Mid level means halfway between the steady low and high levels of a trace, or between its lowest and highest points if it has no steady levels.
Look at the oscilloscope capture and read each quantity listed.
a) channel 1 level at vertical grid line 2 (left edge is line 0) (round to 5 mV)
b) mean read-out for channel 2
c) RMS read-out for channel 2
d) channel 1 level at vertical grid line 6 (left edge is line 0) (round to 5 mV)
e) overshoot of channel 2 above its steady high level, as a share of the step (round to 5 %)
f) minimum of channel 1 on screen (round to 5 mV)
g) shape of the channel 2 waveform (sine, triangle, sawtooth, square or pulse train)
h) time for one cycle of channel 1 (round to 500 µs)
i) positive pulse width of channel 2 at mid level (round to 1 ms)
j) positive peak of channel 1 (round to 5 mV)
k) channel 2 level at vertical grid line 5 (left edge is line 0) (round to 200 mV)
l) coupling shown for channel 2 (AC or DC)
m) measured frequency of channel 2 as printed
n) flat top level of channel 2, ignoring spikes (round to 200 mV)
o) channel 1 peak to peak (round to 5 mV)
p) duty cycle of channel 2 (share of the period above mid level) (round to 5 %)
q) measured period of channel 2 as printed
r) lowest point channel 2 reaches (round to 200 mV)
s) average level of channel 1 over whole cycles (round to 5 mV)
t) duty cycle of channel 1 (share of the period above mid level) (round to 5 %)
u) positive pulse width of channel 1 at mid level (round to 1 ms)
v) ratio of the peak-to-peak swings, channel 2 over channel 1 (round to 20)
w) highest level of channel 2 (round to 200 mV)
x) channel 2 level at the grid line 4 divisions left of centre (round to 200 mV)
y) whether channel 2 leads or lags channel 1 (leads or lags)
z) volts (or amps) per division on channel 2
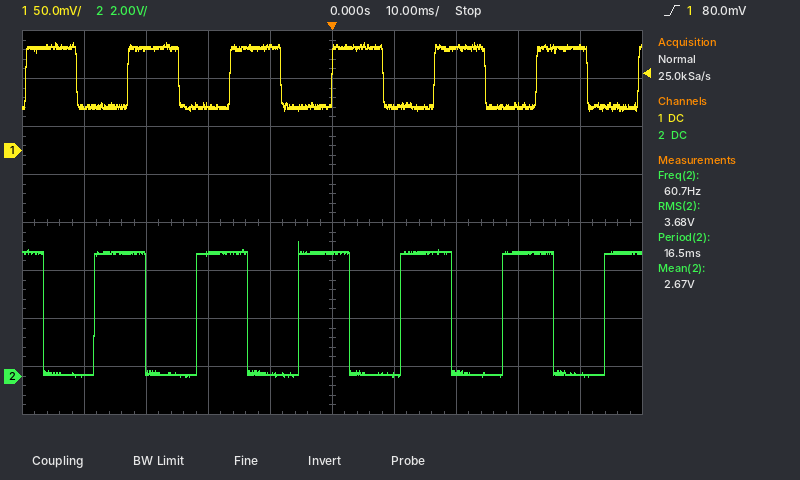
105 mV
2.67 V
3.68 V
45 mV
10 %
40 mV
square
16.5 ms
8 ms
110 mV
5.2 V
DC
60.7 Hz
5.2 V
70 mV
50 %
16.5 ms
0.0 V
75 mV
50 %
8 ms
80
5.6 V
0.0 V
leads
2 V
